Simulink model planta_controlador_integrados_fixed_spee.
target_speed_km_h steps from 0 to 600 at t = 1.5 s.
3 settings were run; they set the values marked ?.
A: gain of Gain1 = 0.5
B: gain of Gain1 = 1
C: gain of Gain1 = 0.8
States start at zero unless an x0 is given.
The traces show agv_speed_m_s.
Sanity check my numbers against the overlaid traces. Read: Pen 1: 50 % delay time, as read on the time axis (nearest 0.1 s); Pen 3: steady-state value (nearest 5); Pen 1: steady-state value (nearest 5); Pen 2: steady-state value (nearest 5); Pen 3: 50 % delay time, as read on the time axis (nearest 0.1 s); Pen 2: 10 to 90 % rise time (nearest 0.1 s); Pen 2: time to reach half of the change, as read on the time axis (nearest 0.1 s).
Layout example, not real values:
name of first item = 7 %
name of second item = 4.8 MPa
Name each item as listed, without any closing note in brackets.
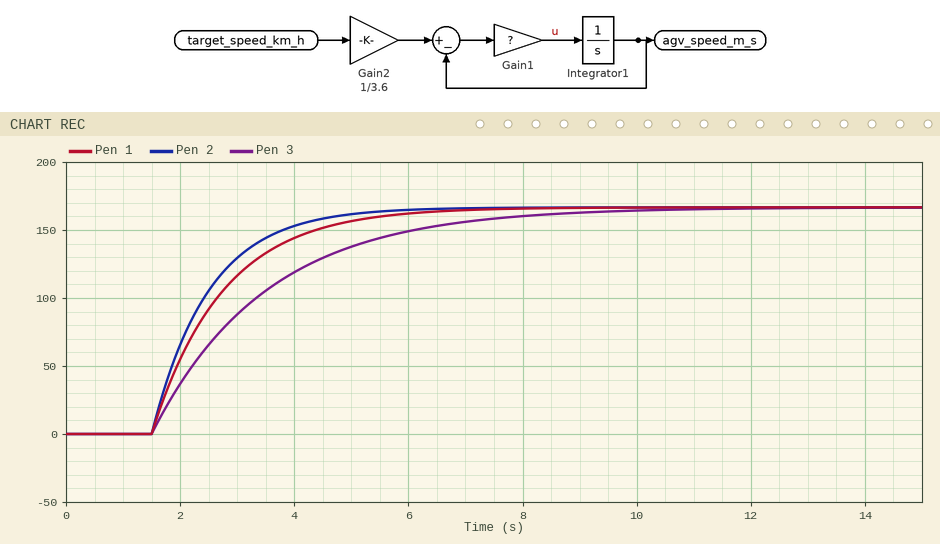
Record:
Pen 1: 50 % delay time, as read on the time axis = 2.4 s
Pen 3: steady-state value = 165
Pen 1: steady-state value = 165
Pen 2: steady-state value = 165
Pen 3: 50 % delay time, as read on the time axis = 2.9 s
Pen 2: 10 to 90 % rise time = 2.2 s
Pen 2: time to reach half of the change, as read on the time axis = 2.2 s
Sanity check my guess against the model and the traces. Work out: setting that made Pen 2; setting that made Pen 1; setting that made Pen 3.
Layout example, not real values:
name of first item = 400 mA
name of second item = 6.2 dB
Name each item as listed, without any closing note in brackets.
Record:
setting that made Pen 2 = B
setting that made Pen 1 = C
setting that made Pen 3 = A
